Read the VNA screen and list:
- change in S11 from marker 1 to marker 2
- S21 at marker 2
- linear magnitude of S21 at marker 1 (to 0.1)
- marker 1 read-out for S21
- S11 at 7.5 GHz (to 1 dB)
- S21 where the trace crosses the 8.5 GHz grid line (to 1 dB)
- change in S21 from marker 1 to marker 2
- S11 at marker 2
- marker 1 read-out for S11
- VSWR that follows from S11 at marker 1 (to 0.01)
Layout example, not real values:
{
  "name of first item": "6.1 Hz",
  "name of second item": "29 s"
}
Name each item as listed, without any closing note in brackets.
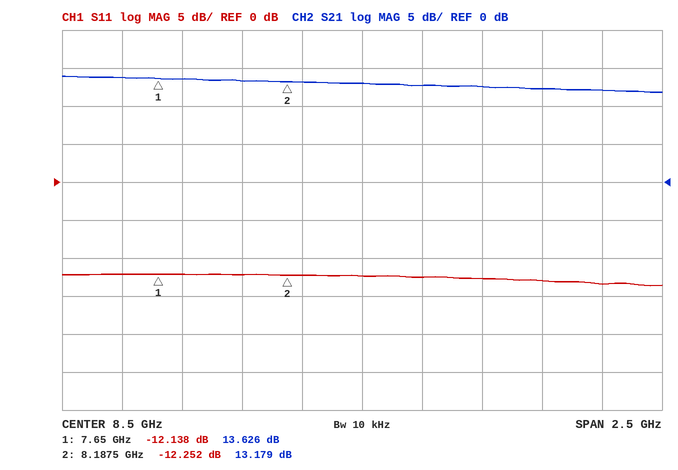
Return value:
{
  "change in S11 from marker 1 to marker 2": "-0.114 dB",
  "S21 at marker 2": "13.179 dB",
  "linear magnitude of S21 at marker 1": "4.8",
  "marker 1 read-out for S21": "13.626 dB",
  "S11 at 7.5 GHz": "-12 dB",
  "S21 where the trace crosses the 8.5 GHz grid line": "13 dB",
  "change in S21 from marker 1 to marker 2": "-0.447 dB",
  "S11 at marker 2": "-12.252 dB",
  "marker 1 read-out for S11": "-12.138 dB",
  "VSWR that follows from S11 at marker 1": "1.66"
}
